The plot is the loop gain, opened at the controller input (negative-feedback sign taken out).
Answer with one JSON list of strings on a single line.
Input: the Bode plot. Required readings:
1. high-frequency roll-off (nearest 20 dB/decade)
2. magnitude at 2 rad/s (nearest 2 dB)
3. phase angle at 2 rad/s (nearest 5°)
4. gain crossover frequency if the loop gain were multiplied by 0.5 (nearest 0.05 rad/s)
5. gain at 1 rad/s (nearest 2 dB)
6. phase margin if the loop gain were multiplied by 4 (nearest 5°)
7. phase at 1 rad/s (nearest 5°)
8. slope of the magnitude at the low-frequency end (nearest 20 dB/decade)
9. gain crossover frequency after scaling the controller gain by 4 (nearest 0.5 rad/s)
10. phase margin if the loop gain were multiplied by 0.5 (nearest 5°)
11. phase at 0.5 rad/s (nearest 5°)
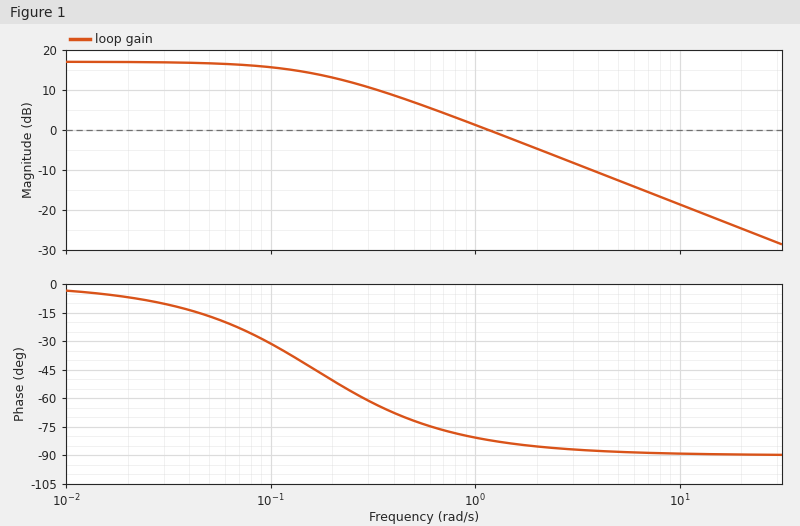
["-20 dB/decade", "-4 dB", "-85°", "0.55 rad/s", "2 dB", "90°", "-80°", "0 dB/decade", "4.5 rad/s", "105°", "-70°"]
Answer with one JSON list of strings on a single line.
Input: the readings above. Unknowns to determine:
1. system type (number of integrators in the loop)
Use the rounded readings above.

["0"]
